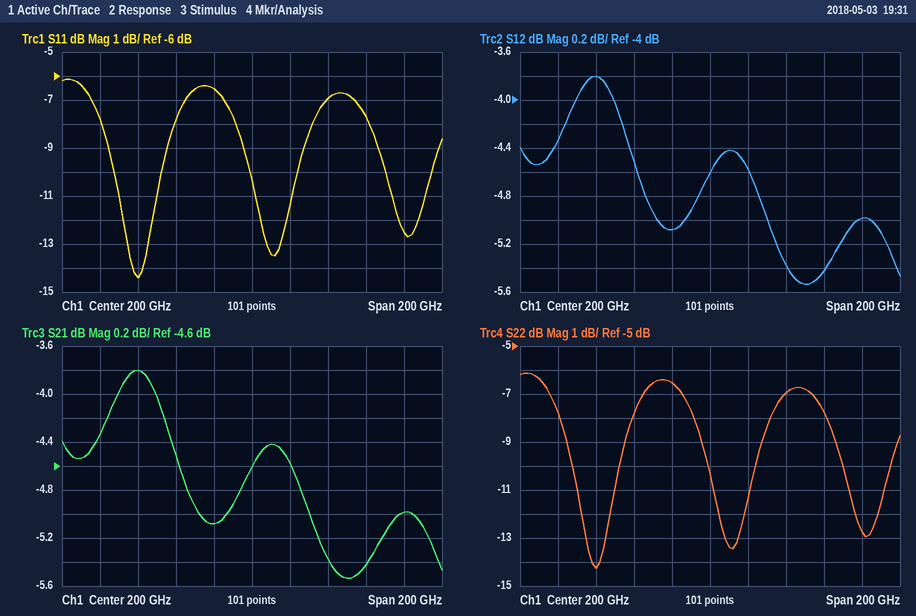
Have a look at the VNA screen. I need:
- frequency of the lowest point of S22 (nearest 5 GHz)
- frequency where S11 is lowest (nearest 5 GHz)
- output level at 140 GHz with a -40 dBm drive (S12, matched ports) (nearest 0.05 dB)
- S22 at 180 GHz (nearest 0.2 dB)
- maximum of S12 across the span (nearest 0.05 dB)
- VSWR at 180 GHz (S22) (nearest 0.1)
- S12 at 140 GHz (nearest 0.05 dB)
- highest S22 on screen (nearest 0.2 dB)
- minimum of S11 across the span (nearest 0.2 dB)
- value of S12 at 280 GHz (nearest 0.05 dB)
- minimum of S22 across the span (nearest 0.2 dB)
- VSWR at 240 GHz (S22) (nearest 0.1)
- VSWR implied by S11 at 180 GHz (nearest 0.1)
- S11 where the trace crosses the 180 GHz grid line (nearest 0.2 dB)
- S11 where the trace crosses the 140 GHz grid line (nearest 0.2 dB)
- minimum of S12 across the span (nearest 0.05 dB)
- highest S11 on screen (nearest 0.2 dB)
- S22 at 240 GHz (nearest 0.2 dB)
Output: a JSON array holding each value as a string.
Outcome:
["140 GHz", "140 GHz", "-43.80 dBm", "-6.6 dB", "-3.80 dB", "2.8", "-3.80 dB", "-6.2 dB", "-14.4 dB", "-5.00 dB", "-14.2 dB", "2.6", "2.8", "-6.6 dB", "-14.4 dB", "-5.55 dB", "-6.2 dB", "-7.0 dB"]
